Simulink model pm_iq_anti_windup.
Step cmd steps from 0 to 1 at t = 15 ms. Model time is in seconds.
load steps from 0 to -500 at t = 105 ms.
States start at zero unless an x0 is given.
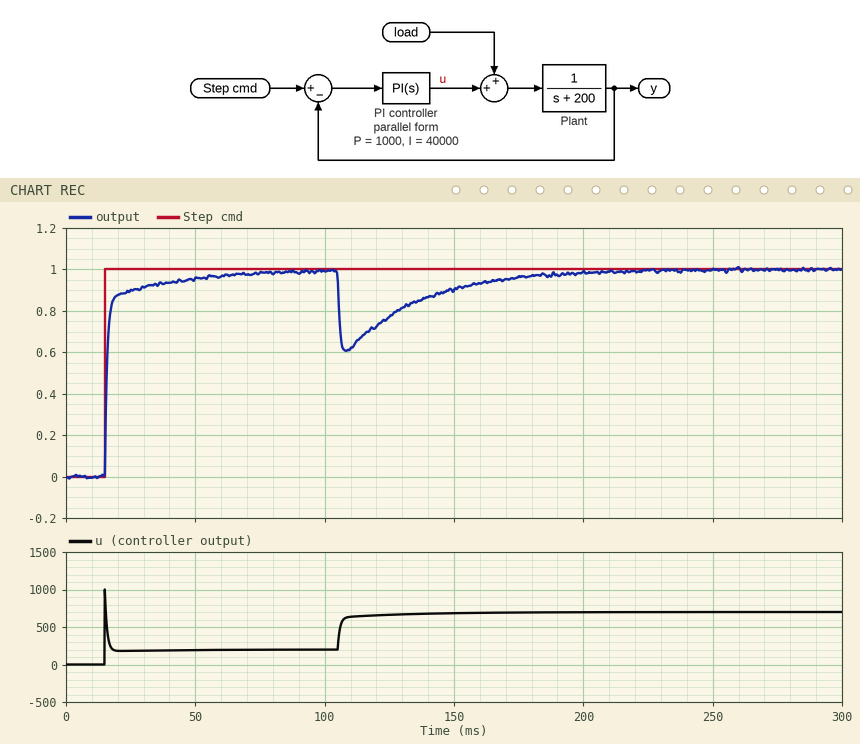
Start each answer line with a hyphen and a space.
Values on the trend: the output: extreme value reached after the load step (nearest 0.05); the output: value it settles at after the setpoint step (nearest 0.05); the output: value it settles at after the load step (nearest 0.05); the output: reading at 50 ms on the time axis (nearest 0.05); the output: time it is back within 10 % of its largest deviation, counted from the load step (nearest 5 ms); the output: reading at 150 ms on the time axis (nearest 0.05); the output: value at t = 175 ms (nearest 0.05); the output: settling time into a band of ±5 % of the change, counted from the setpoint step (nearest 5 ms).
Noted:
- 0.60
- 1.00
- 1.00
- 0.95
- 70 ms
- 0.90
- 0.95
- 30 ms
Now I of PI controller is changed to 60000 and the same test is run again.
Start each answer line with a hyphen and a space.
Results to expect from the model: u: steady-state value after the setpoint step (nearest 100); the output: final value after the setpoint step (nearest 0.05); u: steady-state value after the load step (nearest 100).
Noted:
- 200
- 1.00
- 700
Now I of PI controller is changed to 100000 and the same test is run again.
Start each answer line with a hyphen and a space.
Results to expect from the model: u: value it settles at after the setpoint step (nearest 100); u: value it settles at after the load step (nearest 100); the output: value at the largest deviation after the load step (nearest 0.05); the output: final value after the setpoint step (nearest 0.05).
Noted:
- 200
- 700
- 0.65
- 1.00
